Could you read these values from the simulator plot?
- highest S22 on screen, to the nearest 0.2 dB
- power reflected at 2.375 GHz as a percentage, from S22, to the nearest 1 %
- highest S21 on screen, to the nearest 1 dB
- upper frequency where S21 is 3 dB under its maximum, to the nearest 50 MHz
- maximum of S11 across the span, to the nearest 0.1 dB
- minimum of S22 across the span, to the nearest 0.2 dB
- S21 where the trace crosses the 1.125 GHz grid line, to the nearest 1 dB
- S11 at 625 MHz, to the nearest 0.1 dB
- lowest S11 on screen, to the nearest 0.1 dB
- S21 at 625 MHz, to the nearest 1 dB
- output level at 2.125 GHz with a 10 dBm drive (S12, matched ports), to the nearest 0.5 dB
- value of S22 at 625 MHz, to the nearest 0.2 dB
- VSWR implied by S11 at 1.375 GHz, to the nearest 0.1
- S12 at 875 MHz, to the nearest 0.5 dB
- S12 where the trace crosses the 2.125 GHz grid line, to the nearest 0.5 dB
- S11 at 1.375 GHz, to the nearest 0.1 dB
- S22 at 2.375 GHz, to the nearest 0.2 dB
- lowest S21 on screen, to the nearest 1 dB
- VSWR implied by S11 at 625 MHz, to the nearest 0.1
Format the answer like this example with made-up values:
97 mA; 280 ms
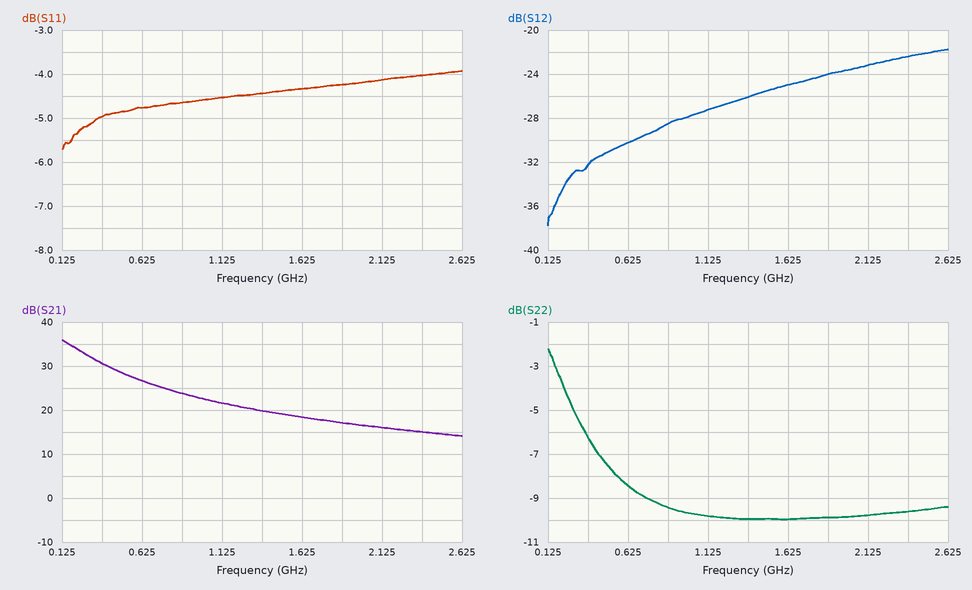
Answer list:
-2.2 dB; 11 %; 36 dB; 250 MHz; -3.9 dB; -10.0 dB; 22 dB; -4.8 dB; -5.7 dB; 27 dB; -13.0 dBm; -8.4 dB; 4.0; -28.5 dB; -23.0 dB; -4.4 dB; -9.6 dB; 14 dB; 3.7
